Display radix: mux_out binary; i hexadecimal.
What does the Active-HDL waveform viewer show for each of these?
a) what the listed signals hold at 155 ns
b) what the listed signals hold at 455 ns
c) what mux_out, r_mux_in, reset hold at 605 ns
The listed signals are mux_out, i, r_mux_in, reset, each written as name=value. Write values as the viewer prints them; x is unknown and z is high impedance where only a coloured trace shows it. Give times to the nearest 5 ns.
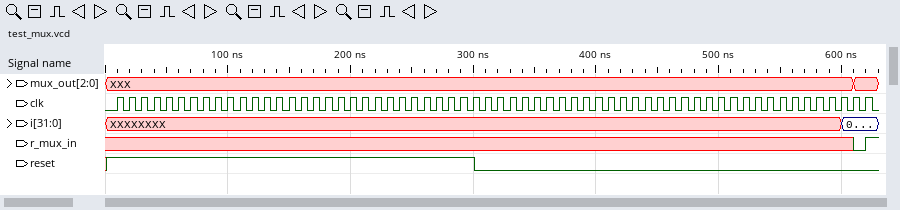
mux_out=XXX, i=XXXXXXXX, r_mux_in=x, reset=1
mux_out=XXX, i=XXXXXXXX, r_mux_in=x, reset=0
mux_out=XXX, r_mux_in=x, reset=0
